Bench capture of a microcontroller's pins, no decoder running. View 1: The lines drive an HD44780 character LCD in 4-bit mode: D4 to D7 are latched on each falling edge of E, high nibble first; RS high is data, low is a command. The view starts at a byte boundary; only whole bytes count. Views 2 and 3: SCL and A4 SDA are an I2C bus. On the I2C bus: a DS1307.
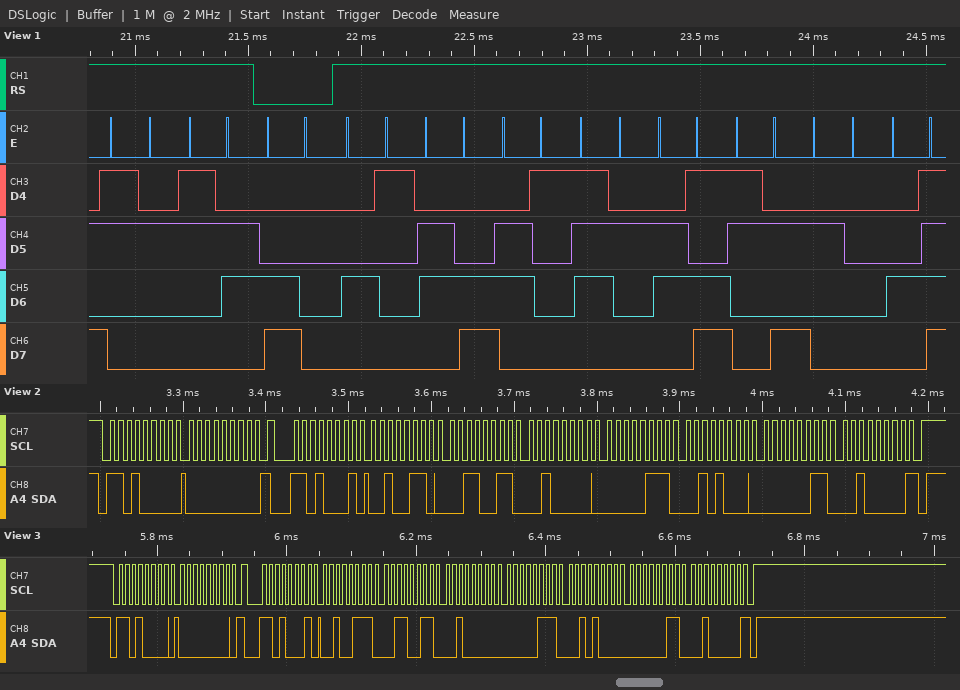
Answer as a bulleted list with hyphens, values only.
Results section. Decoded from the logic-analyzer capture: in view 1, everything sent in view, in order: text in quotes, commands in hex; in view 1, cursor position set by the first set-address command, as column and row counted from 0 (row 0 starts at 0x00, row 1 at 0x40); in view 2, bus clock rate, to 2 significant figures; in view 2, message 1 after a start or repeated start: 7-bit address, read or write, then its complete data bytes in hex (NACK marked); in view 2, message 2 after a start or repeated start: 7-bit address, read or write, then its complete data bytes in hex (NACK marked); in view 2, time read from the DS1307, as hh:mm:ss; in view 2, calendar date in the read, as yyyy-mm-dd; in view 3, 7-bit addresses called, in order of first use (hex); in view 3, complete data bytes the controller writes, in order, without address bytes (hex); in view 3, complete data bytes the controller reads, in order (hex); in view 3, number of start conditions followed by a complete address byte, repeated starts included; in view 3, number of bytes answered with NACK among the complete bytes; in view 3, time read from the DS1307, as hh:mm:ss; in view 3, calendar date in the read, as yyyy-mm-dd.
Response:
- "26" 0xC0 "Alarm: O"
- column 0, row 1
- 100 kHz
- 0x68 write: 00
- 0x68 read: 26 33 20 07 28 03 20 NACK
- 20:33:26
- 2020-03-28
- 0x68
- 00
- 27 33 20 07 28 03 20
- 2
- 1
- 20:33:27
- 2020-03-28
